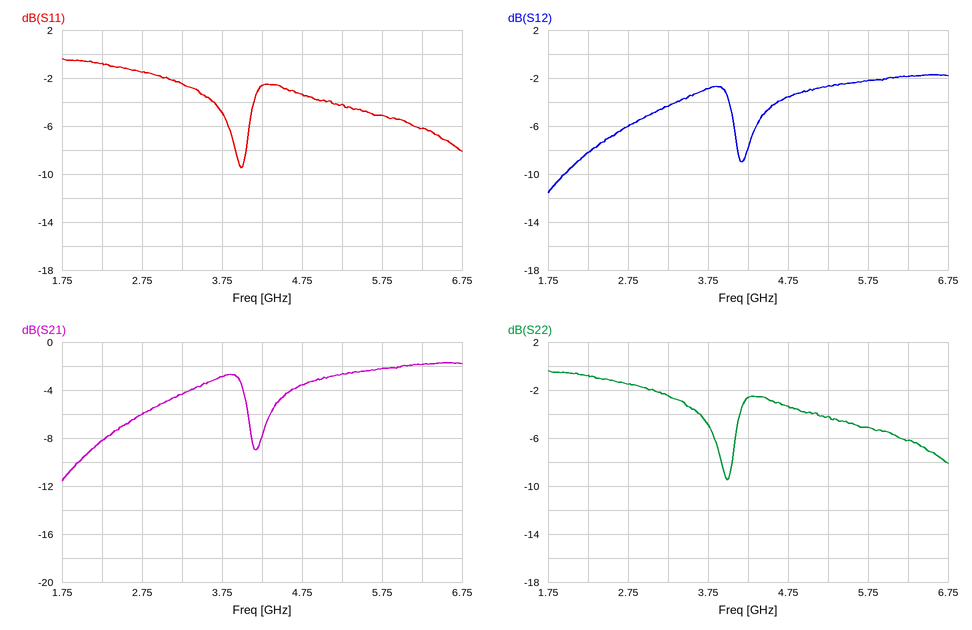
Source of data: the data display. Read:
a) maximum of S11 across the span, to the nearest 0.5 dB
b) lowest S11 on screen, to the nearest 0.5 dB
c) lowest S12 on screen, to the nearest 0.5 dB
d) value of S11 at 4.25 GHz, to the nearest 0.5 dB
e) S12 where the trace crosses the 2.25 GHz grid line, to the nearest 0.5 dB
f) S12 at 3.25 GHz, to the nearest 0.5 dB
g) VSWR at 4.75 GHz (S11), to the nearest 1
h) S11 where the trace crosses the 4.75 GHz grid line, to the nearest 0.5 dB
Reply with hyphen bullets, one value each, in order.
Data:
- -0.5 dB
- -9.5 dB
- -11.5 dB
- -2.5 dB
- -8.0 dB
- -4.5 dB
- 5
- -3.5 dB
